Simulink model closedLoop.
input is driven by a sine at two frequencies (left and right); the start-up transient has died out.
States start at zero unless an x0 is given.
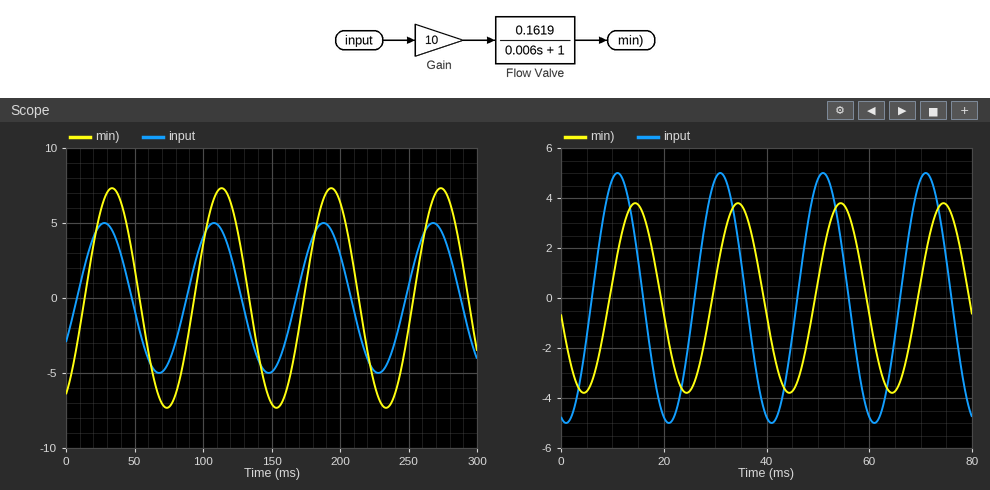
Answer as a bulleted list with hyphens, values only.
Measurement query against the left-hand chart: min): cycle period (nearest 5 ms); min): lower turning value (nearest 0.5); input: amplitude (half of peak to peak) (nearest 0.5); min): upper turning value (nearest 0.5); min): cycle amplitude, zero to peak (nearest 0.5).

- 80 ms
- -7.5
- 5.0
- 7.5
- 7.5
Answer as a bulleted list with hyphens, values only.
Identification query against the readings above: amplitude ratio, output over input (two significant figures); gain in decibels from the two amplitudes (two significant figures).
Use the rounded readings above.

- 1.5
- 3.5 dB
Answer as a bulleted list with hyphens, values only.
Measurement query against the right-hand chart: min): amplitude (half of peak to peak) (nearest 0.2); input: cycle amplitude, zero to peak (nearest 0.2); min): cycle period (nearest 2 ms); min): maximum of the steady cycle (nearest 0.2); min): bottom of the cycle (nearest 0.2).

- 3.8
- 5.0
- 20 ms
- 3.8
- -3.8
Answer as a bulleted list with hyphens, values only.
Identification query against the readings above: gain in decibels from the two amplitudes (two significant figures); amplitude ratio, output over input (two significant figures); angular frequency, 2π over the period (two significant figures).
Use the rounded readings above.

- -2.4 dB
- 0.76
- 0.31 rad/ms
